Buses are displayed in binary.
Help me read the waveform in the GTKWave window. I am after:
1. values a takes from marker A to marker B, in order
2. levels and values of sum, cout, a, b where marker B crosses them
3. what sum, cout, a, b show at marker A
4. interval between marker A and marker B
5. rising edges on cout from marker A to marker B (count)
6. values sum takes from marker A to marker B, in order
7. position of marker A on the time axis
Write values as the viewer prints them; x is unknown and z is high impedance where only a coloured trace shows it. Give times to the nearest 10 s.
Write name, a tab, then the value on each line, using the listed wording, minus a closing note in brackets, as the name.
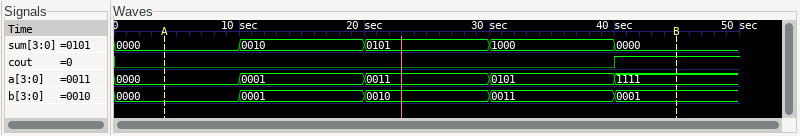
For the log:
values a takes from marker A to marker B, in order	0000, 0001, 0011, 0101, 1111
levels and values of sum, cout, a, b where marker B crosses them	sum=0000, cout=1, a=1111, b=0001
what sum, cout, a, b show at marker A	sum=0000, cout=0, a=0000, b=0000
interval between marker A and marker B	40 s
rising edges on cout from marker A to marker B	1
values sum takes from marker A to marker B, in order	0000, 0010, 0101, 1000, 0000
position of marker A on the time axis	0 s
